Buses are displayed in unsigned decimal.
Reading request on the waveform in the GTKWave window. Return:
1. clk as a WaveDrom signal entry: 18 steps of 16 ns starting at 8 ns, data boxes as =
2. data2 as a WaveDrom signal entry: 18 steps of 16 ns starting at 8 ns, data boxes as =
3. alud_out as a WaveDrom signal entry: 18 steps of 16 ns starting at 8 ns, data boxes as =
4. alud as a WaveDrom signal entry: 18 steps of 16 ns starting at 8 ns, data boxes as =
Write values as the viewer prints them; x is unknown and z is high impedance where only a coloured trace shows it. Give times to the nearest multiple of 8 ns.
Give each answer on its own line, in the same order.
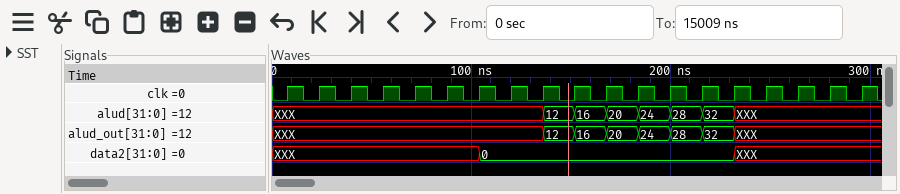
{name: 'clk', wave: 'p.................'}
{name: 'data2', wave: 'x.....=.......x...', data: '0'}
{name: 'alud_out', wave: 'x.......======x...', data: '12 16 20 24 28 32'}
{name: 'alud', wave: 'x.......======x...', data: '12 16 20 24 28 32'}
